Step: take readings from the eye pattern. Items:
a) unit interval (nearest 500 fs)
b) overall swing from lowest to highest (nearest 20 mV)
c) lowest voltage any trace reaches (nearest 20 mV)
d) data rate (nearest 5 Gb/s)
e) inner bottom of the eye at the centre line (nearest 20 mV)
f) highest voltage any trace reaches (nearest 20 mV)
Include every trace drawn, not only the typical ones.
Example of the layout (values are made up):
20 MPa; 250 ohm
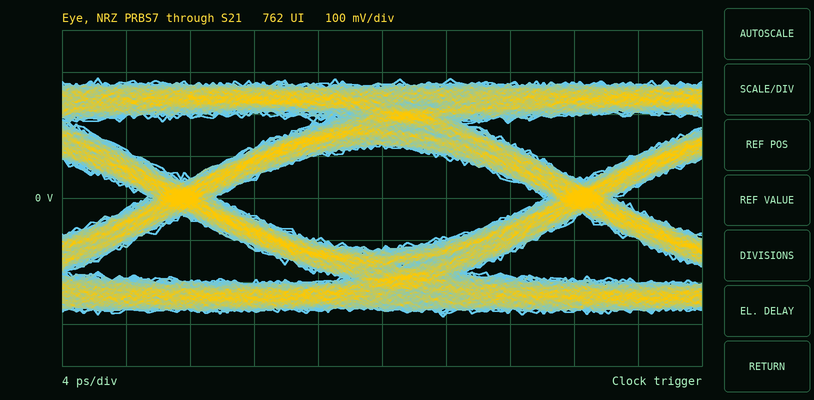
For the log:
25.0 ps; 560 mV; -280 mV; 40 Gb/s; -120 mV; 280 mV
